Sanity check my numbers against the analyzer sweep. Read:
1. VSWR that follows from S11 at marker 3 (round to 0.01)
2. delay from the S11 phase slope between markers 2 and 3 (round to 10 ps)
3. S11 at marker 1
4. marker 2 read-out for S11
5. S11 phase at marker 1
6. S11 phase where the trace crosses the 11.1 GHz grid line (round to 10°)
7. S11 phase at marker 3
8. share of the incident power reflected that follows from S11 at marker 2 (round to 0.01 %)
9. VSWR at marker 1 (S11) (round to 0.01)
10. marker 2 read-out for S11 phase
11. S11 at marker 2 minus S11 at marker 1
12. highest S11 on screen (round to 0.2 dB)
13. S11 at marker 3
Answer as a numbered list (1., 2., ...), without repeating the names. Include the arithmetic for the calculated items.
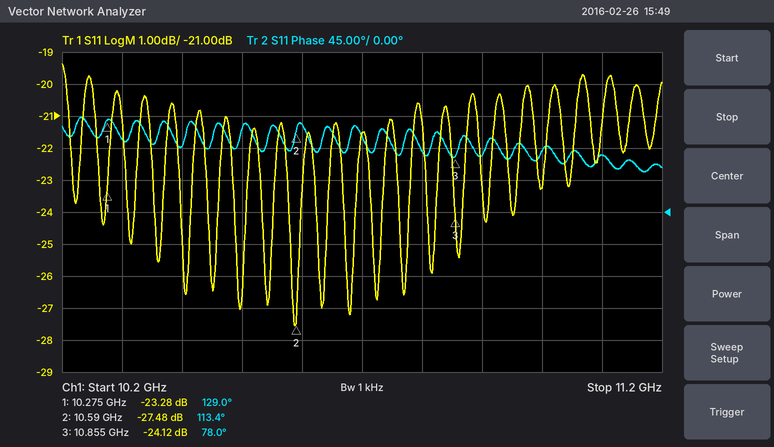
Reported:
1. (1 + 0.0622)/(1 − 0.0622) ≈ 1.13
2. −(78° − (113.4°))/(360° × 265 MHz) ≈ 371 ps, so 370 ps to the nearest 10 ps
3. -23.28 dB
4. -27.48 dB
5. 129.0°
6. 80°
7. 78.0°
8. 10^(-27.48/10) ≈ 0.18 %
9. (1 + 0.0685)/(1 − 0.0685) ≈ 1.15
10. 113.4°
11. -27.48 − (-23.28) = -4.20 dB
12. -19.4 dB
13. -24.12 dB
